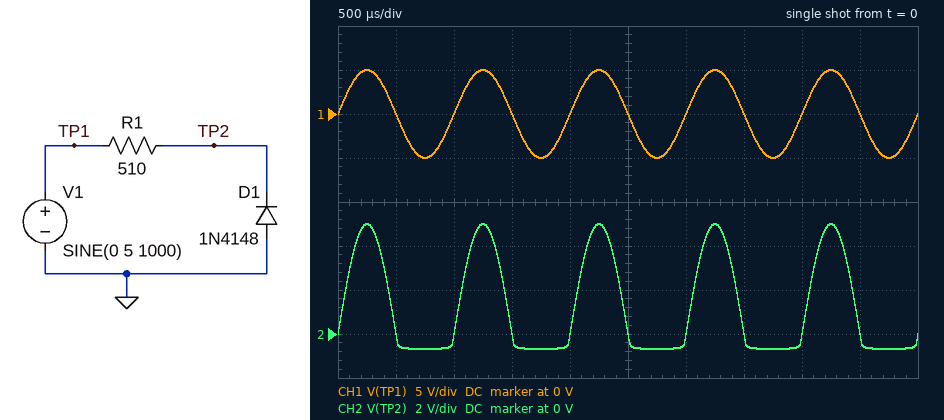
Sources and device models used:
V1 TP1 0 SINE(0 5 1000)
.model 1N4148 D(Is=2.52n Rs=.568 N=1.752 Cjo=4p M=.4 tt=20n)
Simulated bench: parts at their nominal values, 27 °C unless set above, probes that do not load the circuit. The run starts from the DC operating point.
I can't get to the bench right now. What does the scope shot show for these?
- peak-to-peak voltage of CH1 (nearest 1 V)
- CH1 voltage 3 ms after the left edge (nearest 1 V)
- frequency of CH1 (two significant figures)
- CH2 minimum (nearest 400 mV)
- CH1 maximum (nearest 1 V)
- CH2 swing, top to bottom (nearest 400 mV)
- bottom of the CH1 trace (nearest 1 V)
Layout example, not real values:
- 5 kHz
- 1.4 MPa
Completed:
- 10 V
- 0 V
- 1.0 kHz
- -800 mV
- 5 V
- 5.6 V
- -5 V
